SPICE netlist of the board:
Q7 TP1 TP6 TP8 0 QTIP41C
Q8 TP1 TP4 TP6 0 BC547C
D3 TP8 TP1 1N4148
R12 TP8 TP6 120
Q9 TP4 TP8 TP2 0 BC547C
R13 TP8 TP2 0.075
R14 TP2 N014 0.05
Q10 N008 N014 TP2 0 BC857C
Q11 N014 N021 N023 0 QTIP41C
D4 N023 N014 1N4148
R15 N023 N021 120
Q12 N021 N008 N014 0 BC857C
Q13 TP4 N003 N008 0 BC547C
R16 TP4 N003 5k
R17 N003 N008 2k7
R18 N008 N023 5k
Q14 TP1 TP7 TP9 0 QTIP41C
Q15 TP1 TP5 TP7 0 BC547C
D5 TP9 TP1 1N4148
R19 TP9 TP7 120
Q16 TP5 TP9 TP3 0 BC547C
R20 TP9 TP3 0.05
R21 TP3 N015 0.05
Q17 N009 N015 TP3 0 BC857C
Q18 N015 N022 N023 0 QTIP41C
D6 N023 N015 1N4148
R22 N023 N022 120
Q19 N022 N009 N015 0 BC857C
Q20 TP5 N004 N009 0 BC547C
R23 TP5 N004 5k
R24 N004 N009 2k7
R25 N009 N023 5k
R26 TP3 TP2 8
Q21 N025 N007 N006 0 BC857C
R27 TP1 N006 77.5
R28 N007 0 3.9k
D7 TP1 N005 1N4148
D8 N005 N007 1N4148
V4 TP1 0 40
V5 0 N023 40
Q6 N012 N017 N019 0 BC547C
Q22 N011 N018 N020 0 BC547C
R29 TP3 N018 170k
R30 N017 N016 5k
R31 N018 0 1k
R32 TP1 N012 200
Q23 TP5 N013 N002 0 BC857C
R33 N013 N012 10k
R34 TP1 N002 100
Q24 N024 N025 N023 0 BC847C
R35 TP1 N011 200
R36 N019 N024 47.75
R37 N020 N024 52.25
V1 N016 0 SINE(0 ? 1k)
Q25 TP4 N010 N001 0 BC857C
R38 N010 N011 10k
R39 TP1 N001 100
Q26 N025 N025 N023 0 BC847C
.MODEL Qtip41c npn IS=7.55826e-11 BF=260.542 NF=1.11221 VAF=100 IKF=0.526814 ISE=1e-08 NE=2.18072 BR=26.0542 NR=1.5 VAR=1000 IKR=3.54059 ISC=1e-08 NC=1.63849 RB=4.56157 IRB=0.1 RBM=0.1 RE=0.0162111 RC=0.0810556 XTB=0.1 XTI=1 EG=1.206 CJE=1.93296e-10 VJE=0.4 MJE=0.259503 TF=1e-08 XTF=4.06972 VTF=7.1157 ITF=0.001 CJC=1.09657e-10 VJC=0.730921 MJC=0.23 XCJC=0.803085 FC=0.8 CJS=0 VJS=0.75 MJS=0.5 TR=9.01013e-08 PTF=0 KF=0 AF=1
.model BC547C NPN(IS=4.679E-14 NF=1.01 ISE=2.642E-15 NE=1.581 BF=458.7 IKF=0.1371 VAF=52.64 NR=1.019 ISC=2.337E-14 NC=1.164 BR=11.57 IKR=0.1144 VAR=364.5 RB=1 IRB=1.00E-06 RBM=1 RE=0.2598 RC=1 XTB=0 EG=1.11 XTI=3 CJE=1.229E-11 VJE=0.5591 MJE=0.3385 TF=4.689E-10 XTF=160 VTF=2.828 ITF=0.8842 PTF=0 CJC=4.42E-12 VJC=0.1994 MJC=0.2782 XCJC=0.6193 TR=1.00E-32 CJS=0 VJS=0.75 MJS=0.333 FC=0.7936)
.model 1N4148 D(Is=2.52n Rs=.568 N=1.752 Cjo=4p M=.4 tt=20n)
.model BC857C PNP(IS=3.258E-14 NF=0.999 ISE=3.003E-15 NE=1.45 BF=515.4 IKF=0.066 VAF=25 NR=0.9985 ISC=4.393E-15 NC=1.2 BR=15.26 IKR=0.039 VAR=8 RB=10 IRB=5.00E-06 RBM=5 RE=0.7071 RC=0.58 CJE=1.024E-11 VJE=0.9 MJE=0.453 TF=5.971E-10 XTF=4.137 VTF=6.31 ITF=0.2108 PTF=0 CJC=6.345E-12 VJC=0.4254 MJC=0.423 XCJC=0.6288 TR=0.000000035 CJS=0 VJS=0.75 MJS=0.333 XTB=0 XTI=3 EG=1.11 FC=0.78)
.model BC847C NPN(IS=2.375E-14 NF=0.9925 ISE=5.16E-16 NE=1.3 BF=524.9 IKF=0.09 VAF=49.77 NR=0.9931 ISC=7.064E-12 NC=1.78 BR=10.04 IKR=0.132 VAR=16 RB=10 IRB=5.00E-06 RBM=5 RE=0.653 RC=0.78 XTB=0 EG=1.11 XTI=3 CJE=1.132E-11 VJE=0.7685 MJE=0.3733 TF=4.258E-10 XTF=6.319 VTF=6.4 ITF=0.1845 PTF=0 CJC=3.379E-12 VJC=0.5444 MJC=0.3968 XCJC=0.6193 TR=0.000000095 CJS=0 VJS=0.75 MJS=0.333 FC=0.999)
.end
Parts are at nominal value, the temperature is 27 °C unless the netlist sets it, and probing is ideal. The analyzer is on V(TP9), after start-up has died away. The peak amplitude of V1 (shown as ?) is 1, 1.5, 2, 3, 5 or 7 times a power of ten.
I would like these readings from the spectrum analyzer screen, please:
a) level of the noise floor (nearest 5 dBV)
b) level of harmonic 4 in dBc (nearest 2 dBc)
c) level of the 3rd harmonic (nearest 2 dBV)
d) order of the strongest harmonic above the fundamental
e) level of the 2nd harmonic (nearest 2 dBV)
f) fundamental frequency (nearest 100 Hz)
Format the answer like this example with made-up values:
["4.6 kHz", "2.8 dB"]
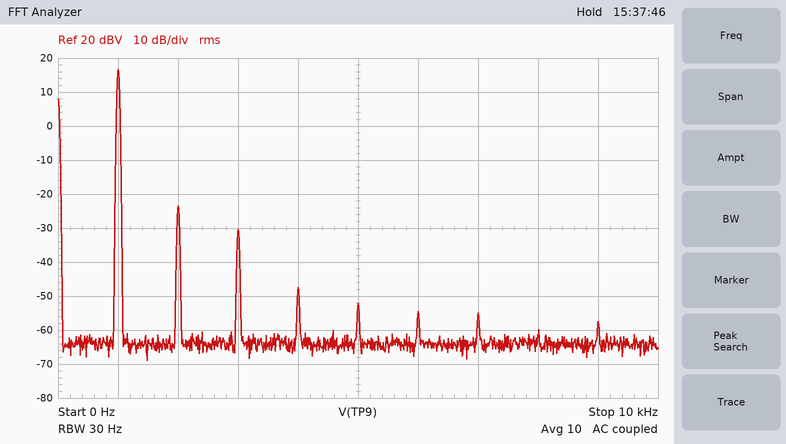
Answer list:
["-65 dBV", "-64 dBc", "-30 dBV", "2", "-24 dBV", "1.0 kHz"]
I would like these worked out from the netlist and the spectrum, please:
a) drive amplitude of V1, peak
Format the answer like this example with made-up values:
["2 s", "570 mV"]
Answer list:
["200 mV"]
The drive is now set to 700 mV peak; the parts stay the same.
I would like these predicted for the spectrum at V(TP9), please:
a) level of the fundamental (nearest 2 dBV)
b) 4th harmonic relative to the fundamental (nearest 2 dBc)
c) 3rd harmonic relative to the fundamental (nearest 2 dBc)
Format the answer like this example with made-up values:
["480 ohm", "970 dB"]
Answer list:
["26 dBV", "-38 dBc", "-24 dBc"]
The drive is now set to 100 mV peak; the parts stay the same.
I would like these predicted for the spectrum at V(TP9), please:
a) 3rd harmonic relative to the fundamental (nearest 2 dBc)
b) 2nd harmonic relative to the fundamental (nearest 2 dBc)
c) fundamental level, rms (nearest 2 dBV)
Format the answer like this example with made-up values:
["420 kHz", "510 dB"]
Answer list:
["-54 dBc", "-44 dBc", "10 dBV"]
